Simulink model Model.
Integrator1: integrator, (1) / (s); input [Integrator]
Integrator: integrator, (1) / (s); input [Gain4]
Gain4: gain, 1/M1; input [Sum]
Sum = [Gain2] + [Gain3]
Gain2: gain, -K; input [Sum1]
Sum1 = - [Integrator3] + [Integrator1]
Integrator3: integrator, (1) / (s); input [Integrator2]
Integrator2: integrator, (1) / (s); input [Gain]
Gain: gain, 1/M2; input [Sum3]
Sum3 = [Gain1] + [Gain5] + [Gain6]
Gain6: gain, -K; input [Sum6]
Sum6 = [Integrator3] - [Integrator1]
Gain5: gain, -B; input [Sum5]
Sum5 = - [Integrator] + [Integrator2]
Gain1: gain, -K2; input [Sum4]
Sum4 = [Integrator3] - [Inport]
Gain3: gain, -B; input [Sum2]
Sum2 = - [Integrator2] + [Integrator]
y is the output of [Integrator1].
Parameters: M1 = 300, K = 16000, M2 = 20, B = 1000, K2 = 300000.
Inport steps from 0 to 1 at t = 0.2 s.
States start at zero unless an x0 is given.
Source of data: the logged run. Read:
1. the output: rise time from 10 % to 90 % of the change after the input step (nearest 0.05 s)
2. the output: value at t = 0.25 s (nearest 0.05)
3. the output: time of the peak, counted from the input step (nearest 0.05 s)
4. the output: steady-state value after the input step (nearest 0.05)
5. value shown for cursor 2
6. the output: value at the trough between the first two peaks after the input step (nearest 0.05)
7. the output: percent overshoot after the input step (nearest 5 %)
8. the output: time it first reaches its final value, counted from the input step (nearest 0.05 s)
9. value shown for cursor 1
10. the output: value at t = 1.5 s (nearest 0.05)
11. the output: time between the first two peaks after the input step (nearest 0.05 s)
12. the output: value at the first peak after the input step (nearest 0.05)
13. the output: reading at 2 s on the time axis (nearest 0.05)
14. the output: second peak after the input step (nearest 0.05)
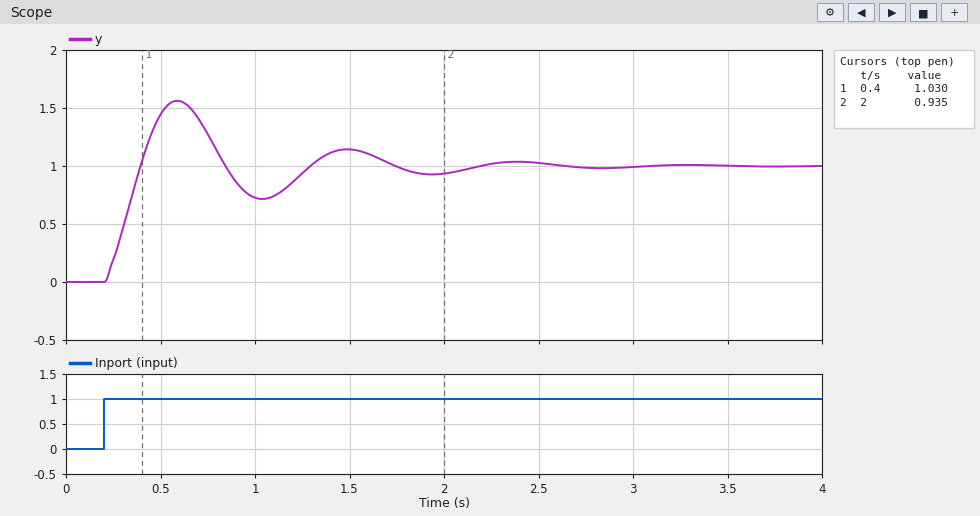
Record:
0.15 s
0.20
0.40 s
1.00
0.935
0.70
55 %
0.20 s
1.030
1.15
0.90 s
1.55
0.95
1.15
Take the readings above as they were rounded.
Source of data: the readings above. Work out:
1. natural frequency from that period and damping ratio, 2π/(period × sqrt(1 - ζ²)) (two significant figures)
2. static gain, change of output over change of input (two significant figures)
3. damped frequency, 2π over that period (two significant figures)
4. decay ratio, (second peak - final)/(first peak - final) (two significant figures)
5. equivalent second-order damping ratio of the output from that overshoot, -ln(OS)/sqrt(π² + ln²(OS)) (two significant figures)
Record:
7.1 rad/s
1.0
7.0 rad/s
0.27
0.19
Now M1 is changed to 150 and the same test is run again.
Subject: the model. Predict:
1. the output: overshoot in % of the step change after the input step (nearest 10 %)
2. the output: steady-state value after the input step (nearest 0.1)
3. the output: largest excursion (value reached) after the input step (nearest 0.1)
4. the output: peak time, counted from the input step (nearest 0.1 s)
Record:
50 %
1.0
1.5
0.3 s
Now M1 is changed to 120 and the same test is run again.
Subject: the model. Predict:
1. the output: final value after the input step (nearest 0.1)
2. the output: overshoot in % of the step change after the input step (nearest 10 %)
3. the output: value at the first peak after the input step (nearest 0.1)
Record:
1.0
40 %
1.4
